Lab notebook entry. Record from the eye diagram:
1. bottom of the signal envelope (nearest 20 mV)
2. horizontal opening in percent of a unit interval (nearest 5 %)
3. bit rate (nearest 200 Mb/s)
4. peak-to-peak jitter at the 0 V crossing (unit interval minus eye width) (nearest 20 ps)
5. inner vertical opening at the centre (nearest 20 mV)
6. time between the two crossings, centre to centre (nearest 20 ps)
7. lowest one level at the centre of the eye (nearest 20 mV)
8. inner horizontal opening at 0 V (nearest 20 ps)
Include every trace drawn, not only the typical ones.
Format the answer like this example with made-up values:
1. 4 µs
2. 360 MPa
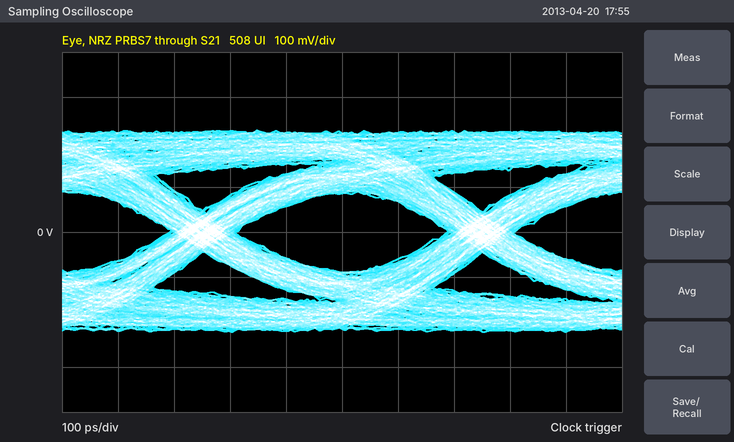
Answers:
1. -220 mV
2. 75 %
3. 2.0 Gb/s
4. 120 ps
5. 180 mV
6. 500 ps
7. 80 mV
8. 380 ps
